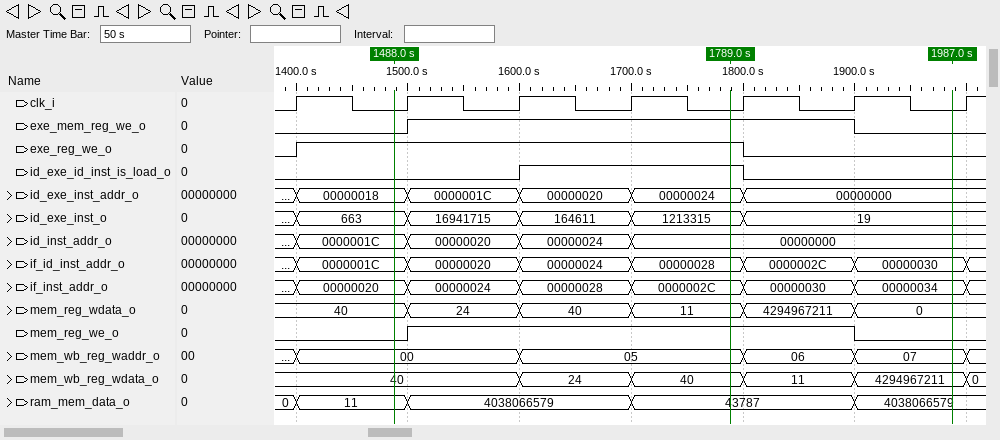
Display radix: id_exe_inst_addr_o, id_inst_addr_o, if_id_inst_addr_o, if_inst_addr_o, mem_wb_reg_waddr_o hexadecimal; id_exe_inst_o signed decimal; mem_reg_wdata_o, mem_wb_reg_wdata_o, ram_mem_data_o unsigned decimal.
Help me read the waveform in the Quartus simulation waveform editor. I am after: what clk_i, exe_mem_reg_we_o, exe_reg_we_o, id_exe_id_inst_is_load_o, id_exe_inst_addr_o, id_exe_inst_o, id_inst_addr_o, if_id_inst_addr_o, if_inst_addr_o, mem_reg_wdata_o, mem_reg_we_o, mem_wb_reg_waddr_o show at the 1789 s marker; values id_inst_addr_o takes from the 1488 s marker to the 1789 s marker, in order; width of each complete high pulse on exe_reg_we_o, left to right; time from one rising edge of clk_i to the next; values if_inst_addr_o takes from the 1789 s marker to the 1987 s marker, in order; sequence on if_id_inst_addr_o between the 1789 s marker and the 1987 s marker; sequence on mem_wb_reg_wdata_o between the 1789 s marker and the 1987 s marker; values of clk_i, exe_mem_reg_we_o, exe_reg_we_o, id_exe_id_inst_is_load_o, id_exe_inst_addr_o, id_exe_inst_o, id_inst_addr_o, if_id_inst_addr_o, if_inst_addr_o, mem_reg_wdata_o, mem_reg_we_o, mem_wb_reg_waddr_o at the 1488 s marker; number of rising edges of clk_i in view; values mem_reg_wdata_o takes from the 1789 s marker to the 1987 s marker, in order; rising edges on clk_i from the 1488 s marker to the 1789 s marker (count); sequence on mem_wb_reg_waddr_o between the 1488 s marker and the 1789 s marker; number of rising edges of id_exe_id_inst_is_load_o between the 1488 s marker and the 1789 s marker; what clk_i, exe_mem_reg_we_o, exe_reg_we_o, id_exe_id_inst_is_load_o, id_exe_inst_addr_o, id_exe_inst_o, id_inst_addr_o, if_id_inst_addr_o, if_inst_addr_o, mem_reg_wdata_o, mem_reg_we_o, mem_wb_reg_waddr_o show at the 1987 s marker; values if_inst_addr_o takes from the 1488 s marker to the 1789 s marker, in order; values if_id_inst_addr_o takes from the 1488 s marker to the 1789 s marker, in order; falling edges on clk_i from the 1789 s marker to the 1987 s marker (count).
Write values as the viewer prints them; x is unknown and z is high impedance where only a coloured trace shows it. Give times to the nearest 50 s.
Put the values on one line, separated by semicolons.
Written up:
clk_i=0, exe_mem_reg_we_o=1, exe_reg_we_o=1, id_exe_id_inst_is_load_o=1, id_exe_inst_addr_o=00000024, id_exe_inst_o=1213315, id_inst_addr_o=00000000, if_id_inst_addr_o=00000028, if_inst_addr_o=0000002C, mem_reg_wdata_o=11, mem_reg_we_o=1, mem_wb_reg_waddr_o=05; 0000001C, 00000020, 00000024, 00000000; 400 s; 100 s; 0000002C, 00000030, 00000034; 00000028, 0000002C, 00000030; 40, 11, 4294967211; clk_i=0, exe_mem_reg_we_o=0, exe_reg_we_o=1, id_exe_id_inst_is_load_o=0, id_exe_inst_addr_o=00000018, id_exe_inst_o=663, id_inst_addr_o=0000001C, if_id_inst_addr_o=0000001C, if_inst_addr_o=00000020, mem_reg_wdata_o=40, mem_reg_we_o=0, mem_wb_reg_waddr_o=00; 7; 11, 4294967211, 0; 3; 00, 05; 1; clk_i=0, exe_mem_reg_we_o=0, exe_reg_we_o=0, id_exe_id_inst_is_load_o=0, id_exe_inst_addr_o=00000000, id_exe_inst_o=19, id_inst_addr_o=00000000, if_id_inst_addr_o=00000030, if_inst_addr_o=00000034, mem_reg_wdata_o=0, mem_reg_we_o=0, mem_wb_reg_waddr_o=07; 00000020, 00000024, 00000028, 0000002C; 0000001C, 00000020, 00000024, 00000028; 2
